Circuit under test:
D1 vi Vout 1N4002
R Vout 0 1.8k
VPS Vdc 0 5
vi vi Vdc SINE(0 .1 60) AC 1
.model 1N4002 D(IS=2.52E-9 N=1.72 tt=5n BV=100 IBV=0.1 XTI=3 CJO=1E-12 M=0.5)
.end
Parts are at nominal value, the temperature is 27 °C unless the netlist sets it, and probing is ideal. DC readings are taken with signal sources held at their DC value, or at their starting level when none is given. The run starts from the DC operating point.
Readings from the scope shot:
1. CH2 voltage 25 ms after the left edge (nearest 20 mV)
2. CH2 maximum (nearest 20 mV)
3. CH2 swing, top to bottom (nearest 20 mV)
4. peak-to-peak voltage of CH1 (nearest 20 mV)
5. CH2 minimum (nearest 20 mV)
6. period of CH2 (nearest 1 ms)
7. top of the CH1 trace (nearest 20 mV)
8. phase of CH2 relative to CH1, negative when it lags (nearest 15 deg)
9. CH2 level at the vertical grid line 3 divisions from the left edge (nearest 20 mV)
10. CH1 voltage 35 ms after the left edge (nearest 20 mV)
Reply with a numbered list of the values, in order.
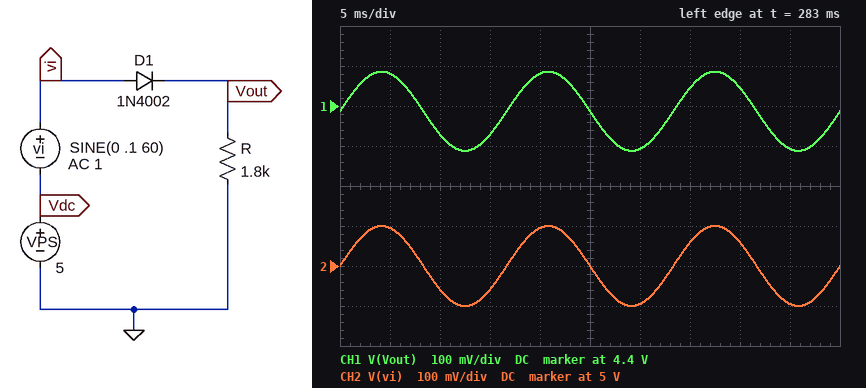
1. 5.00 V
2. 5.10 V
3. 200 mV
4. 200 mV
5. 4.90 V
6. 17 ms
7. 4.48 V
8. 0 deg
9. 4.94 V
10. 4.44 V
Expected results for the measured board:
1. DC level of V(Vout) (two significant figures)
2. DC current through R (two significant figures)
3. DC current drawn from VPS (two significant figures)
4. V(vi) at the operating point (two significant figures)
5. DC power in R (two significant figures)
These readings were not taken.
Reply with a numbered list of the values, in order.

1. 4.4 V
2. 2.4 mA
3. 2.4 mA
4. 5.0 V
5. 11 mW
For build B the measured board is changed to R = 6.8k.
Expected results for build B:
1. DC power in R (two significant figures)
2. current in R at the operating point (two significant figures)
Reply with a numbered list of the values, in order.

1. 2.9 mW
2. 650 µA
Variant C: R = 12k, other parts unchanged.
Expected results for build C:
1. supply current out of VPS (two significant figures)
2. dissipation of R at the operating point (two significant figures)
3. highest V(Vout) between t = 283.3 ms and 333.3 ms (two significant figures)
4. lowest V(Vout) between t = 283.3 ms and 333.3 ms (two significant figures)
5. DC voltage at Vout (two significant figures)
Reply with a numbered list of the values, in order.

1. 370 µA
2. 1.7 mW
3. 4.6 V
4. 4.4 V
5. 4.5 V
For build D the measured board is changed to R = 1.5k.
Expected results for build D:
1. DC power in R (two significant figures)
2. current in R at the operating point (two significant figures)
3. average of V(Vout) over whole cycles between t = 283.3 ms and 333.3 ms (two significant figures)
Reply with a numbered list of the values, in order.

1. 13 mW
2. 2.9 mA
3. 4.4 V
